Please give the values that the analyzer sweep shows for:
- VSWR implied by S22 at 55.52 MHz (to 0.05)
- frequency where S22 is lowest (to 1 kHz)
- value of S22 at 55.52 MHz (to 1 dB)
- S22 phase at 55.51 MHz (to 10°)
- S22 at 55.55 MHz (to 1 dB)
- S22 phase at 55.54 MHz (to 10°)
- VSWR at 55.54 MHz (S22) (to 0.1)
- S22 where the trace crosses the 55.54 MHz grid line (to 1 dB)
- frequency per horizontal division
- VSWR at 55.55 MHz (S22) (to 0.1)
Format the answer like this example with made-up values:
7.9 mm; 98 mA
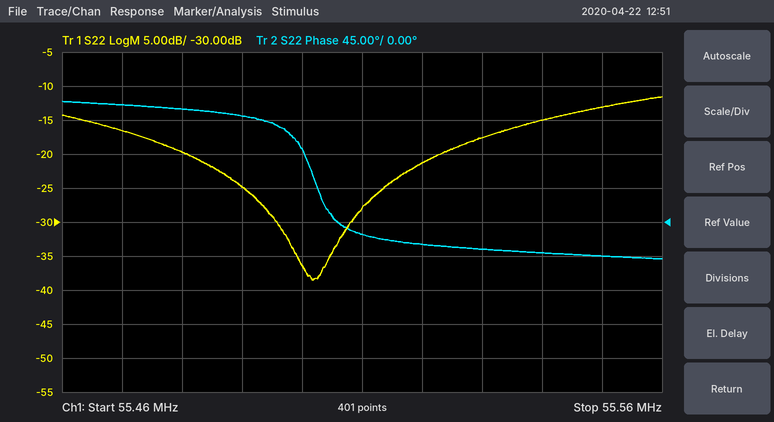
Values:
1.20; 55.502 MHz; -21 dB; -20°; -13 dB; -40°; 1.4; -15 dB; 10 kHz; 1.6
